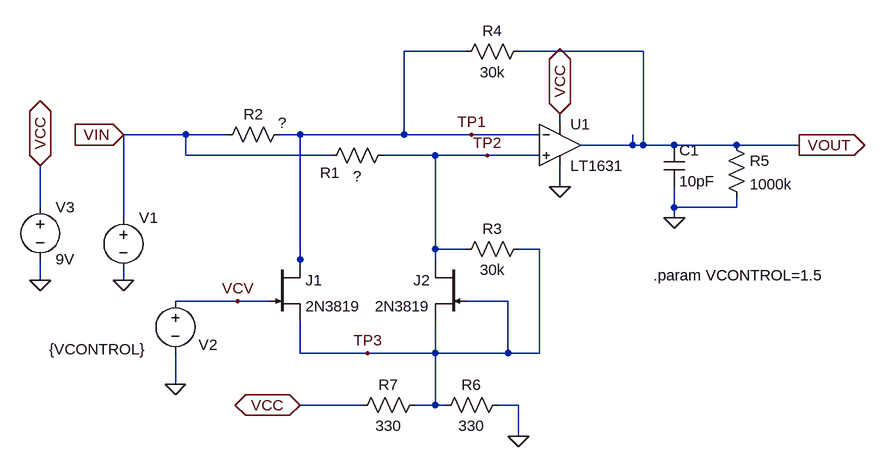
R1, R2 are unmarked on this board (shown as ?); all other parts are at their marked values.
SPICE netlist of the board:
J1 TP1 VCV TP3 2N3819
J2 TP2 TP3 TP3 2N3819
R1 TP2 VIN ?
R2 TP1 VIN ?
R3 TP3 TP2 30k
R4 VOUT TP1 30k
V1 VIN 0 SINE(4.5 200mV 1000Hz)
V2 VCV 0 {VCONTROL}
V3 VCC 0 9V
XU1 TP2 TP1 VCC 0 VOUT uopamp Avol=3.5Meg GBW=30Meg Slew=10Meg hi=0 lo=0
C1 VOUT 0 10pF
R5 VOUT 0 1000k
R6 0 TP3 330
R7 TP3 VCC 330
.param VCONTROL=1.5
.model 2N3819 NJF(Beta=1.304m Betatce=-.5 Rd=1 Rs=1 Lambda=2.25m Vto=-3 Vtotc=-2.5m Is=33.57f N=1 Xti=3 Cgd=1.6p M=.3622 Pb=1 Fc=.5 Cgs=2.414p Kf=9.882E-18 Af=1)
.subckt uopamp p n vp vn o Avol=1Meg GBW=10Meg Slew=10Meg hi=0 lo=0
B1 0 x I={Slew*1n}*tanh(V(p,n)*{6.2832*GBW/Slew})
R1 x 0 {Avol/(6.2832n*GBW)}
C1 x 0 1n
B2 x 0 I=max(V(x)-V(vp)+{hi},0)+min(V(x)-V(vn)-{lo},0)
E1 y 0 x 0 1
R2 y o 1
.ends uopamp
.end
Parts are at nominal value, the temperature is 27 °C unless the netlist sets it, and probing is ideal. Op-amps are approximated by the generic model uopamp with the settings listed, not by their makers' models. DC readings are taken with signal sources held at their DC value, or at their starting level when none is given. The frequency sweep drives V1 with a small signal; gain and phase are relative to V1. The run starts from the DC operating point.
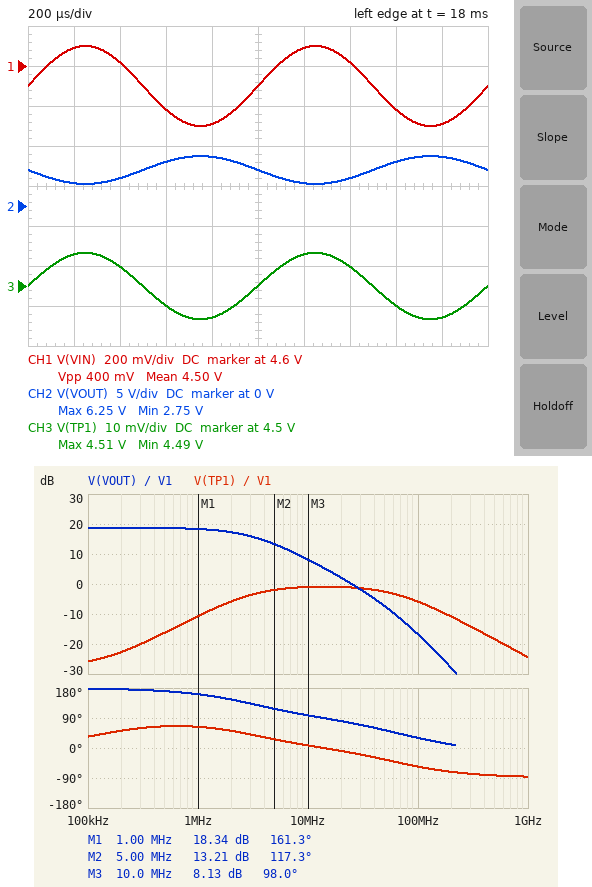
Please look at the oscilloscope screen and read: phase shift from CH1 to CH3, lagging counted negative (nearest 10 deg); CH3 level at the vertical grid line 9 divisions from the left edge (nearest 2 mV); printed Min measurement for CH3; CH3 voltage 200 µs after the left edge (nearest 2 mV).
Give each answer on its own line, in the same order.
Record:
0 deg
4.492 V
4.49 V
4.508 V
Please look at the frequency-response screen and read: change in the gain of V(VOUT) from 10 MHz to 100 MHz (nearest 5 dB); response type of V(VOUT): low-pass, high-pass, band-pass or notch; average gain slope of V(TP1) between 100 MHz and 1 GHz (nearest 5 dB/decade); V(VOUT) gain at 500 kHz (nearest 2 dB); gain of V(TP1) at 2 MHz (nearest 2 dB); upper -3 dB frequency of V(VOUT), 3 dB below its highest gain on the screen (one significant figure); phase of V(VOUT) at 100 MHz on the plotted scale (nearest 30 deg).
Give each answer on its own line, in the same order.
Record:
-25 dB
low-pass
-20 dB/decade
18 dB
-6 dB
3 MHz
30 deg
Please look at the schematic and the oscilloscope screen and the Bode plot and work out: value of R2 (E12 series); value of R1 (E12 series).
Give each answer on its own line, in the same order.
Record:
3.3 kΩ
6.8 kΩ
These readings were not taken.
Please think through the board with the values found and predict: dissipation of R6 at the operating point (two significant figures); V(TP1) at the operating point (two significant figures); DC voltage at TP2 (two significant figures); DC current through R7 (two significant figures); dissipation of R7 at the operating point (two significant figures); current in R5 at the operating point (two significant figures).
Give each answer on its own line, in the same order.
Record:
61 mW
4.5 V
4.5 V
14 mA
61 mW
4.5 µA
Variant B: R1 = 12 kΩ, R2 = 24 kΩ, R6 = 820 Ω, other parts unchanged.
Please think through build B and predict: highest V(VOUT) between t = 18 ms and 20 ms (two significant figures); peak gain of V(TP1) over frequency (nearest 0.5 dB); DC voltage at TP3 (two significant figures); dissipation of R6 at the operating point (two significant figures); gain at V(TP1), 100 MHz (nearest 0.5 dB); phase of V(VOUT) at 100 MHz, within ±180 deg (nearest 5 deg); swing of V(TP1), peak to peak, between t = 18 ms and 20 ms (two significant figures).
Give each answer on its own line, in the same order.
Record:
8.9 V
-5.0 dB
6.4 V
50 mW
-20.0 dB
-5 deg
12 mV
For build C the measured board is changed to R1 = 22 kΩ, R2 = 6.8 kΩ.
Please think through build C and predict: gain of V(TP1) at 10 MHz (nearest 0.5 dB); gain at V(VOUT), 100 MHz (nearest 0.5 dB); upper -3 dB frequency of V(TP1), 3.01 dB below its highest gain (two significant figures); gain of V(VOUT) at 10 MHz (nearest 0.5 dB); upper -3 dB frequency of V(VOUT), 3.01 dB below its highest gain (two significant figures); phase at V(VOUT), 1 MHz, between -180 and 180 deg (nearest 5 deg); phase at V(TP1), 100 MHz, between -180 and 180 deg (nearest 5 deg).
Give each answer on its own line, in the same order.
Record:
-2.0 dB
-21.5 dB
41 MHz
7.5 dB
6.5 MHz
170 deg
-70 deg
